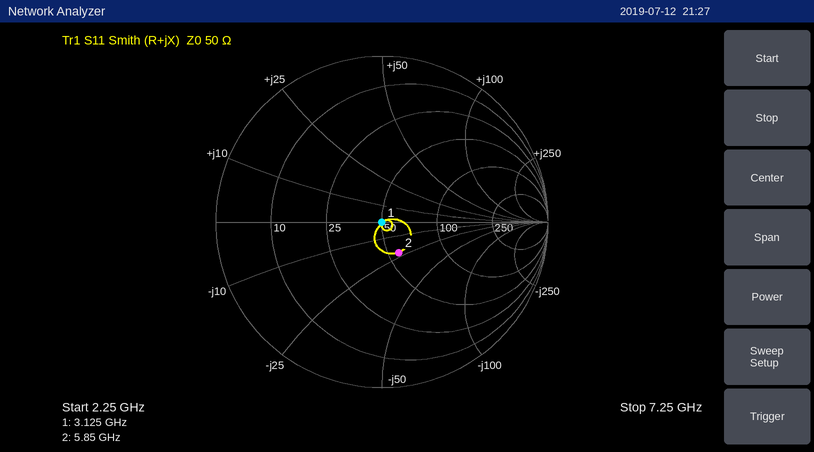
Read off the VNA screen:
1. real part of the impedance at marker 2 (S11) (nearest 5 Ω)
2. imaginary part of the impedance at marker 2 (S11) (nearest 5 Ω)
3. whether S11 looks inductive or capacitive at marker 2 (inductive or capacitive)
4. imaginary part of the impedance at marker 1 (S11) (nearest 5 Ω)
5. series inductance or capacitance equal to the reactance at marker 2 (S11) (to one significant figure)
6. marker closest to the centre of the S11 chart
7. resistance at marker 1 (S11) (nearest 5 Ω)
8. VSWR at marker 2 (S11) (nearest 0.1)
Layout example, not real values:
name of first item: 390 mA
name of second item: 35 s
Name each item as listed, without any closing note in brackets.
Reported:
real part of the impedance at marker 2 (S11): 55 Ω
imaginary part of the impedance at marker 2 (S11): -20 Ω
whether S11 looks inductive or capacitive at marker 2: capacitive
imaginary part of the impedance at marker 1 (S11): 0 Ω
series inductance or capacitance equal to the reactance at marker 2 (S11): 1 pF
marker closest to the centre of the S11 chart: marker 1
resistance at marker 1 (S11): 50 Ω
VSWR at marker 2 (S11): 1.5
